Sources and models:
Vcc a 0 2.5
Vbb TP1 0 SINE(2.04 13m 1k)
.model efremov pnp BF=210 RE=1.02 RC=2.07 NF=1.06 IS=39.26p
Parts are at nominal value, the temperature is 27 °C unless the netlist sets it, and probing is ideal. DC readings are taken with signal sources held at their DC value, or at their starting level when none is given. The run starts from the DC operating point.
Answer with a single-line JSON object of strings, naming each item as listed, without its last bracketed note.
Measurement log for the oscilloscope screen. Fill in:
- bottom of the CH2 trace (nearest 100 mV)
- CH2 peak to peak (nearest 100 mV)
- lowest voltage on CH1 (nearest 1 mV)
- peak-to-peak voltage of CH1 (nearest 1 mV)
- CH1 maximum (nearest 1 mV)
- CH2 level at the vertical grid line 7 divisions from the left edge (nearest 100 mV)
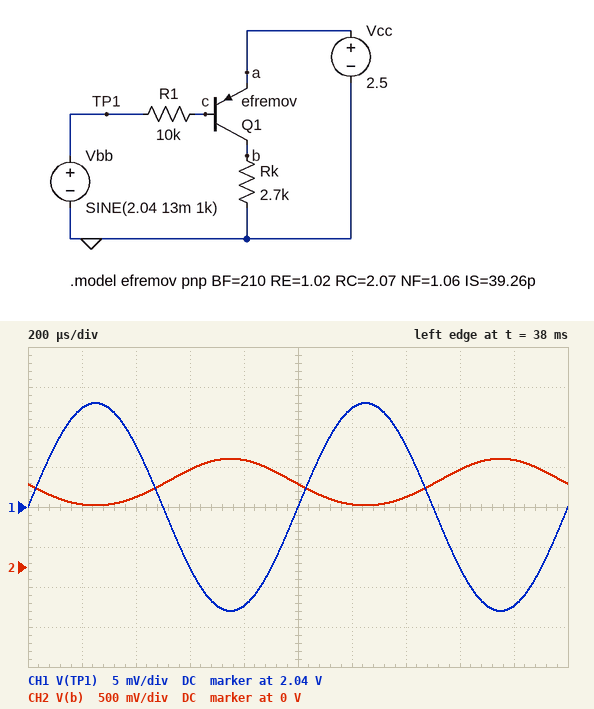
{"bottom of the CH2 trace": "800 mV", "CH2 peak to peak": "600 mV", "lowest voltage on CH1": "2.027 V", "peak-to-peak voltage of CH1": "26 mV", "CH1 maximum": "2.053 V", "CH2 level at the vertical grid line 7 divisions from the left edge": "900 mV"}
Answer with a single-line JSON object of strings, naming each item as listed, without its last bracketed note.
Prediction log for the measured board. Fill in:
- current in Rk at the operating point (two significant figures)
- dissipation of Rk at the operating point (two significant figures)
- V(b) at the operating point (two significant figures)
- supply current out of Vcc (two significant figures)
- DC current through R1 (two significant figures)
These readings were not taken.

{"current in Rk at the operating point": "380 µA", "dissipation of Rk at the operating point": "400 µW", "V(b) at the operating point": "1.0 V", "supply current out of Vcc": "390 µA", "DC current through R1": "1.8 µA"}
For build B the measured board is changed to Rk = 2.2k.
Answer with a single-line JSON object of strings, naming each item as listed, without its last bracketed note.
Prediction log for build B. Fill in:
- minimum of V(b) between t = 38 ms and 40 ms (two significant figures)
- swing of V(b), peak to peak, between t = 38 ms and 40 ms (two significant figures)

{"minimum of V(b) between t = 38 ms and 40 ms": "630 mV", "swing of V(b), peak to peak, between t = 38 ms and 40 ms": "480 mV"}
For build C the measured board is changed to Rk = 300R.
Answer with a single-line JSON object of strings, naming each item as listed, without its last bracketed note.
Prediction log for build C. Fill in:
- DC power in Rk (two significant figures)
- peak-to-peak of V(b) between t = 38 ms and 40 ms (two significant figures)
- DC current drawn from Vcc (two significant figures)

{"DC power in Rk": "44 µW", "peak-to-peak of V(b) between t = 38 ms and 40 ms": "65 mV", "DC current drawn from Vcc": "390 µA"}
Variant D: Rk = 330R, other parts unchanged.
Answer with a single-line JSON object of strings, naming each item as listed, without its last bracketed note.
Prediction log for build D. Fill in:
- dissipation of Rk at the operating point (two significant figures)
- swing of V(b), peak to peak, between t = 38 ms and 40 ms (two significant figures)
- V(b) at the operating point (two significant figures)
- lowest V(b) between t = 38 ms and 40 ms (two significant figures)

{"dissipation of Rk at the operating point": "49 µW", "swing of V(b), peak to peak, between t = 38 ms and 40 ms": "71 mV", "V(b) at the operating point": "130 mV", "lowest V(b) between t = 38 ms and 40 ms": "94 mV"}
